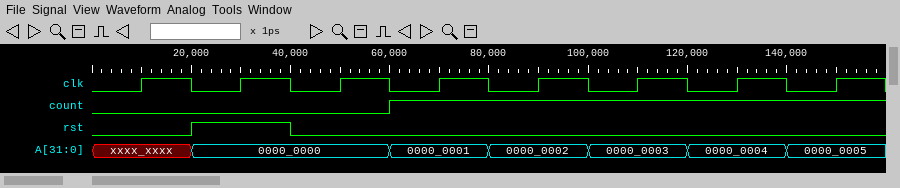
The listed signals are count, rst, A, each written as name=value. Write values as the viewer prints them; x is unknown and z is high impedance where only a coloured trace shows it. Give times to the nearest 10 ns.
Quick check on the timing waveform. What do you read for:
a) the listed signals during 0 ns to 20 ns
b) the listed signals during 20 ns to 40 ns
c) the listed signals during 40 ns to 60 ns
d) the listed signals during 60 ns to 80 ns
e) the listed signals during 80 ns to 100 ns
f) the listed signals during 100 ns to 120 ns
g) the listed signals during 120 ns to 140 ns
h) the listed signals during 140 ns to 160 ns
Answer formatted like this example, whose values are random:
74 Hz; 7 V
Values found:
count=0, rst=0, A=xxxx_xxxx; count=0, rst=1, A=0000_0000; count=0, rst=0, A=0000_0000; count=1, rst=0, A=0000_0001; count=1, rst=0, A=0000_0002; count=1, rst=0, A=0000_0003; count=1, rst=0, A=0000_0004; count=1, rst=0, A=0000_0005
